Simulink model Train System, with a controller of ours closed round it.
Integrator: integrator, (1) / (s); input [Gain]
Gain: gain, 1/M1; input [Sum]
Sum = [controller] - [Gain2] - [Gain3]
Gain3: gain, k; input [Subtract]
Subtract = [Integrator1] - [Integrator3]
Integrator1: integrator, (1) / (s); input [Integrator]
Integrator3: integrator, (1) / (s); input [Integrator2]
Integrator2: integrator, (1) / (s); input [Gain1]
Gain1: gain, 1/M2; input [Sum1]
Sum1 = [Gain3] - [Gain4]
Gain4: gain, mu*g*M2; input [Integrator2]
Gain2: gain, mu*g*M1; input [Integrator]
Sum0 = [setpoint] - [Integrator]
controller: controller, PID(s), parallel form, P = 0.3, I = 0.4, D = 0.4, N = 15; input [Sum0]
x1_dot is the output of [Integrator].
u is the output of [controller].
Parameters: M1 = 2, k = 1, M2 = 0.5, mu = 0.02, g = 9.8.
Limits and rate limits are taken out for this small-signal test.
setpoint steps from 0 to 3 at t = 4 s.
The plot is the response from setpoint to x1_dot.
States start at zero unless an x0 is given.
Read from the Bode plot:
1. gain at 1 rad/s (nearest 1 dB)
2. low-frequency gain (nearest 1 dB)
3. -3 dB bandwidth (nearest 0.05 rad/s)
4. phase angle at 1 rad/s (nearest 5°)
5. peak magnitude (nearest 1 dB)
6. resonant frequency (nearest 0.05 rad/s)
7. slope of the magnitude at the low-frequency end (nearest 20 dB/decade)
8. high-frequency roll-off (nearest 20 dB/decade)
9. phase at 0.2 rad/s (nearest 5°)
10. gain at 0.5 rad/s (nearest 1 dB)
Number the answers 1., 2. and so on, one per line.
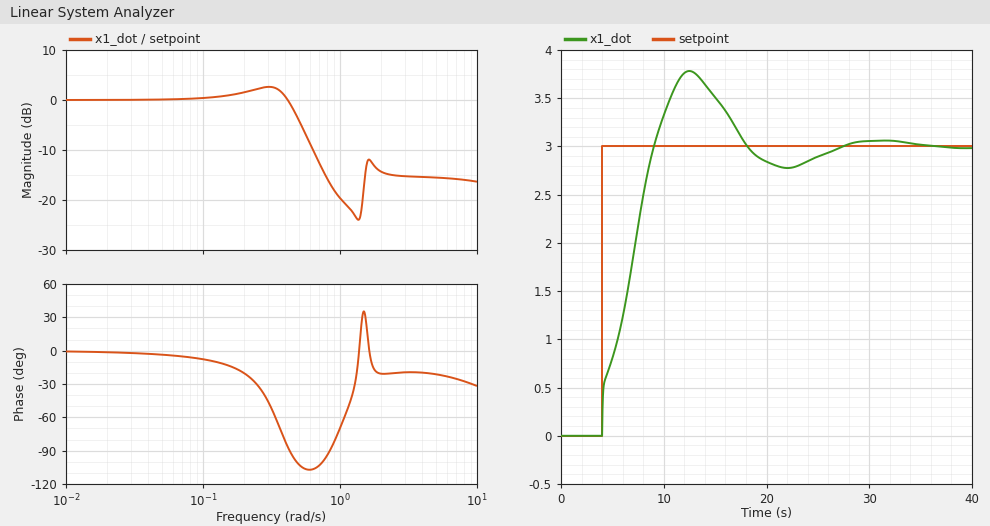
1. -20 dB
2. 0 dB
3. 0.50 rad/s
4. -70°
5. 3 dB
6. 0.30 rad/s
7. 0 dB/decade
8. 0 dB/decade
9. -20°
10. -4 dB
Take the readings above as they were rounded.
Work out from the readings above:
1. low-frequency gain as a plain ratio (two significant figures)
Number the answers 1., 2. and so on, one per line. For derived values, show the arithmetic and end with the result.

1. 10^(0 / 20) = 1.0
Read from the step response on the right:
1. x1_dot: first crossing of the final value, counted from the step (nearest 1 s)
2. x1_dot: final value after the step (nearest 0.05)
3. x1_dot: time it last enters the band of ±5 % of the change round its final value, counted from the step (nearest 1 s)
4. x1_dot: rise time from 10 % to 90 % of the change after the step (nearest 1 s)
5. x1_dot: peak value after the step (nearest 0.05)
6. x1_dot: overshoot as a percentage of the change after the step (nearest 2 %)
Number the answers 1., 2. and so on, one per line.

1. 5 s
2. 3.00
3. 20 s
4. 4 s
5. 3.80
6. 26 %
